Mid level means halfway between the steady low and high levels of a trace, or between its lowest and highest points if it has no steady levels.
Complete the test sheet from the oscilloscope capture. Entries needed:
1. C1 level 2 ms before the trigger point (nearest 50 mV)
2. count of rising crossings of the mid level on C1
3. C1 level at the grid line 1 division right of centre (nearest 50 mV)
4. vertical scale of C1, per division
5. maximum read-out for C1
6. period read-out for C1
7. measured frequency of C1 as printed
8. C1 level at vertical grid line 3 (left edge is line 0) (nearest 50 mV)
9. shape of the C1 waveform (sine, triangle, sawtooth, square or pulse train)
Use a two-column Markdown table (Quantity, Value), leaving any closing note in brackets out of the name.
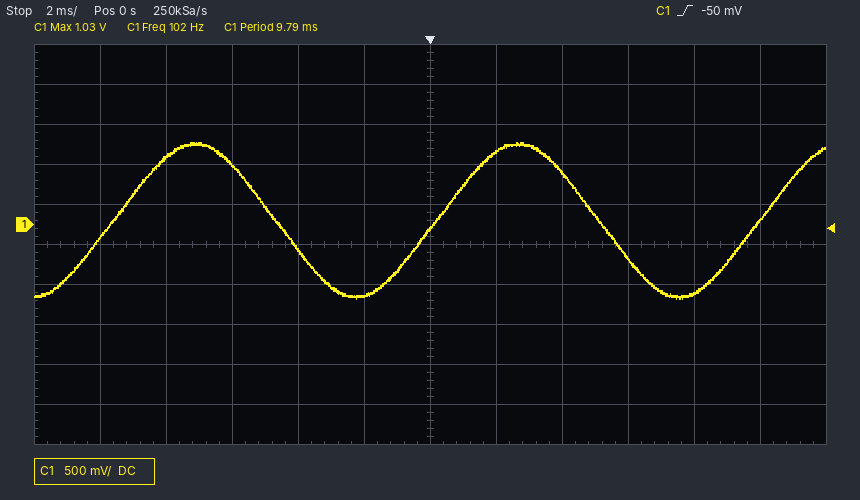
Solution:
| Quantity | Value |
|---|---|
| C1 level 2 ms before the trigger point | -900 mV |
| count of rising crossings of the mid level on C1 | 3 |
| C1 level at the grid line 1 division right of centre | 900 mV |
| vertical scale of C1, per division | 500 mV |
| maximum read-out for C1 | 1.03 V |
| period read-out for C1 | 9.79 ms |
| measured frequency of C1 as printed | 102 Hz |
| C1 level at vertical grid line 3 (left edge is line 0) | 750 mV |
| shape of the C1 waveform | sine |
